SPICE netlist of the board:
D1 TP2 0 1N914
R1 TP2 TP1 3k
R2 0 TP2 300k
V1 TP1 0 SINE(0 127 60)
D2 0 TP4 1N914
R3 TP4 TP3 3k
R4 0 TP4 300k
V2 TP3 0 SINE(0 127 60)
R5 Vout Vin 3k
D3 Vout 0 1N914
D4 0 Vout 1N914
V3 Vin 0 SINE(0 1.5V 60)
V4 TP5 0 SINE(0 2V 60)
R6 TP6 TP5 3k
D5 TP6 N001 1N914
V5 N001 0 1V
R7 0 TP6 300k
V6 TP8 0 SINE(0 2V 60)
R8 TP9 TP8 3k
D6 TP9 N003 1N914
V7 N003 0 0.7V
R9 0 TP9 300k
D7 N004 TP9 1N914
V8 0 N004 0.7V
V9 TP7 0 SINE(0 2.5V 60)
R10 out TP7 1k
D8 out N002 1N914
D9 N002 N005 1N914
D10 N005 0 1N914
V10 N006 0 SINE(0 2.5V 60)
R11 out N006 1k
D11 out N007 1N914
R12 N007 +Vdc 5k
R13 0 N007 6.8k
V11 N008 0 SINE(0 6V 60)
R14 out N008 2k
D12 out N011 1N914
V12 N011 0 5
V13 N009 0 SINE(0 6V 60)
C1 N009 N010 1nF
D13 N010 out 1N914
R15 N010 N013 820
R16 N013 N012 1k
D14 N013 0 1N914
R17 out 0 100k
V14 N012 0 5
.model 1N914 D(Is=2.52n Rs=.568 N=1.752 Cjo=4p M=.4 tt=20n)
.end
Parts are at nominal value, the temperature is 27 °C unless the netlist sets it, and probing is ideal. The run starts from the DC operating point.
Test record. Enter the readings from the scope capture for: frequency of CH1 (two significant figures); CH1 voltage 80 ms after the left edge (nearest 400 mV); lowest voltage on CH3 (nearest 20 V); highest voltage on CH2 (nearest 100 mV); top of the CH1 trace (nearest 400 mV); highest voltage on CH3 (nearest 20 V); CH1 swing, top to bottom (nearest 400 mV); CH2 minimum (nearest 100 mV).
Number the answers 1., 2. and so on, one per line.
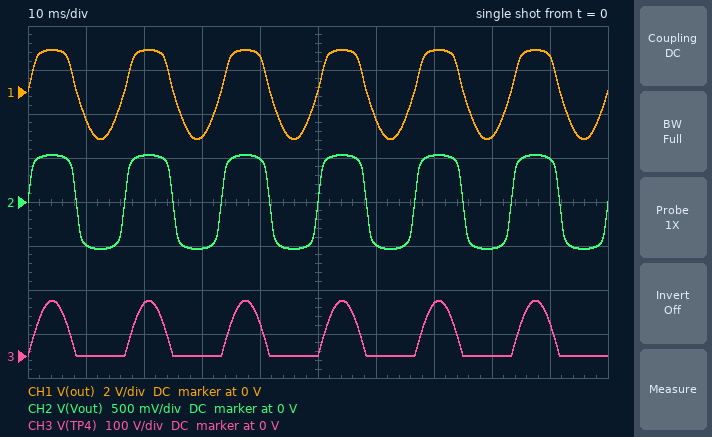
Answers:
1. 60 Hz
2. -2.0 V
3. 0 V
4. 500 mV
5. 2.0 V
6. 120 V
7. 4.0 V
8. -500 mV
